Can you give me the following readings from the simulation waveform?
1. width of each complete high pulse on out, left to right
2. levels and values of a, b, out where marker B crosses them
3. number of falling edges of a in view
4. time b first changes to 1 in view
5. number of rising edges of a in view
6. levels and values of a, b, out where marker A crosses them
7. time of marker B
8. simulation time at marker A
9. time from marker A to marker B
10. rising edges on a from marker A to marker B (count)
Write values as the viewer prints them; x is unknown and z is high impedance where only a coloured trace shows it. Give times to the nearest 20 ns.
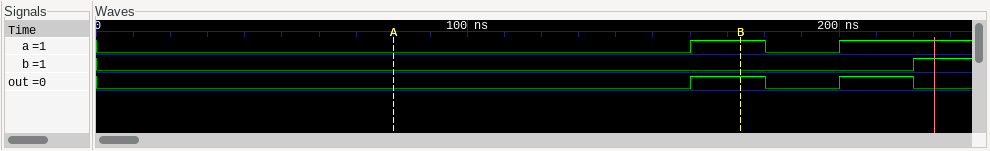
20 ns, 20 ns
a=1, b=0, out=1
1
220 ns
2
a=0, b=0, out=0
180 ns
80 ns
100 ns
1
